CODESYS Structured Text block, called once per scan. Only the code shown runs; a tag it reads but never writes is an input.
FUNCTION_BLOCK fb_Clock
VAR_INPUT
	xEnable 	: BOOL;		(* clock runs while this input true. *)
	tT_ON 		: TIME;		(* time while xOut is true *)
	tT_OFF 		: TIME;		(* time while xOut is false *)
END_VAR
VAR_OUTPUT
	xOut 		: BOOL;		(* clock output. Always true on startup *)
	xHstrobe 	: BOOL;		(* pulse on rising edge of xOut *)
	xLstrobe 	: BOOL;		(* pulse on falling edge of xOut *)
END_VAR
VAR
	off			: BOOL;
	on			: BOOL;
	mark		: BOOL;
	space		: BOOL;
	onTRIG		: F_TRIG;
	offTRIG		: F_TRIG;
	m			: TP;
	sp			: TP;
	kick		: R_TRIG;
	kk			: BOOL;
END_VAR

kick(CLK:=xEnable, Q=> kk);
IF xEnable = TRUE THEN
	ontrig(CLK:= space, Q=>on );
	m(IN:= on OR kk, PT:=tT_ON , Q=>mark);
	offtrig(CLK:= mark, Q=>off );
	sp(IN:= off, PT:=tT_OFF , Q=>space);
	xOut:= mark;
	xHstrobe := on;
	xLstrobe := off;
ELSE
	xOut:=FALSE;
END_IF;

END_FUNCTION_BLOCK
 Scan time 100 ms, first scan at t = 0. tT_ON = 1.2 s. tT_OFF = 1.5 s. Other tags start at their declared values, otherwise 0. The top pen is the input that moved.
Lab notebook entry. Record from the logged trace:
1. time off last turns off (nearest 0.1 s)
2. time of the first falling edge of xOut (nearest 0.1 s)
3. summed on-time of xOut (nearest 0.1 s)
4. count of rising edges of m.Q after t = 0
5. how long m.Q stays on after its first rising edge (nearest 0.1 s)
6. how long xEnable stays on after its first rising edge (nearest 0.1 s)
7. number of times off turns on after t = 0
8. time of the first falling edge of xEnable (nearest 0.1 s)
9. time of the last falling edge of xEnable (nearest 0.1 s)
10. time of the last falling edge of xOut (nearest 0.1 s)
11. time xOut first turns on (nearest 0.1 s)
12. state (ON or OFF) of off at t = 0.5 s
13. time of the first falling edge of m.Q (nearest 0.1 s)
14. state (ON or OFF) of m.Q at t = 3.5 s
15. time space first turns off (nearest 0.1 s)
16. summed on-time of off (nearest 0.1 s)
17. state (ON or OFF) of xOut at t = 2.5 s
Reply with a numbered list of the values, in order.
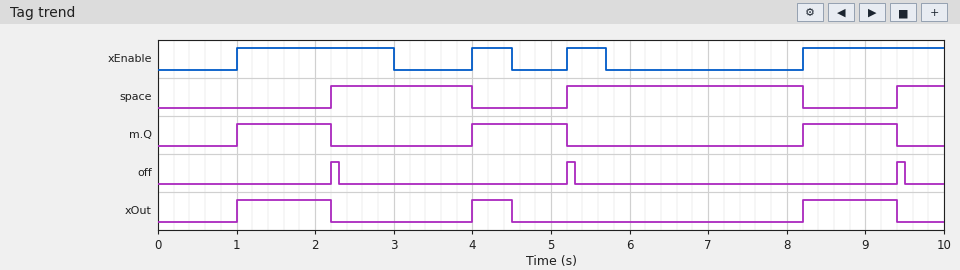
1. 9.5 s
2. 2.2 s
3. 2.9 s
4. 3
5. 1.2 s
6. 2.0 s
7. 3
8. 3.0 s
9. 5.7 s
10. 9.4 s
11. 1.0 s
12. OFF
13. 2.2 s
14. OFF
15. 4.0 s
16. 0.3 s
17. OFF
